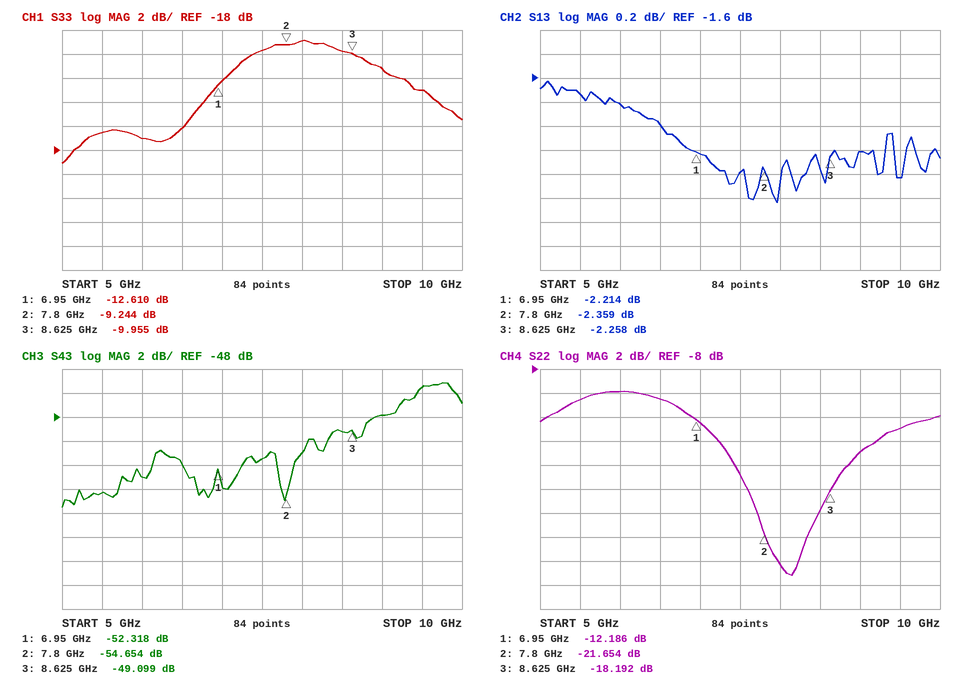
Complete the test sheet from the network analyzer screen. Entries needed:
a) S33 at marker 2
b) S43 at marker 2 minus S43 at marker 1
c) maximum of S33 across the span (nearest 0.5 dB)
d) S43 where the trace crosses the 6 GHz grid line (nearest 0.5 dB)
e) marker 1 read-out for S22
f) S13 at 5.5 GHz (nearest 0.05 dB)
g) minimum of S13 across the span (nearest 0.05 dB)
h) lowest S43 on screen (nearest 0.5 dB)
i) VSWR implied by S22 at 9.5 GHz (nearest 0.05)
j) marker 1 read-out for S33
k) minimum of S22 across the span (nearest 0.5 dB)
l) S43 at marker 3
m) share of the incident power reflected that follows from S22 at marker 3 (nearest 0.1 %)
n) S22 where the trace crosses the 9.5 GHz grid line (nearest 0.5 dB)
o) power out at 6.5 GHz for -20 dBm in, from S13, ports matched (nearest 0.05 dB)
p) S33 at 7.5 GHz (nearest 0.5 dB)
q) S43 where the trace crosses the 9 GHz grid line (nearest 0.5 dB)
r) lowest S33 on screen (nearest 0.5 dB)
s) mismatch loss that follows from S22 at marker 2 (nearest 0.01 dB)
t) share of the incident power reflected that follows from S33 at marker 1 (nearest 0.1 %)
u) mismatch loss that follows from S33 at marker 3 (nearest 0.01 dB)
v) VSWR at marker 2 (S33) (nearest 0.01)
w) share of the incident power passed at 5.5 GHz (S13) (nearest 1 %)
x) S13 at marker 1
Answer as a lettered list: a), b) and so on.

a) -9.244 dB
b) -2.336 dB
c) -9.0 dB
d) -53.0 dB
e) -12.186 dB
f) -1.75 dB
g) -2.65 dB
h) -55.5 dB
i) 1.60
j) -12.610 dB
k) -25.0 dB
l) -49.099 dB
m) 1.5 %
n) -13.0 dB
o) -22.00 dBm
p) -9.5 dB
q) -48.0 dB
r) -19.0 dB
s) 0.03 dB
t) 5.5 %
u) 0.46 dB
v) 2.05
w) 67 %
x) -2.214 dB
